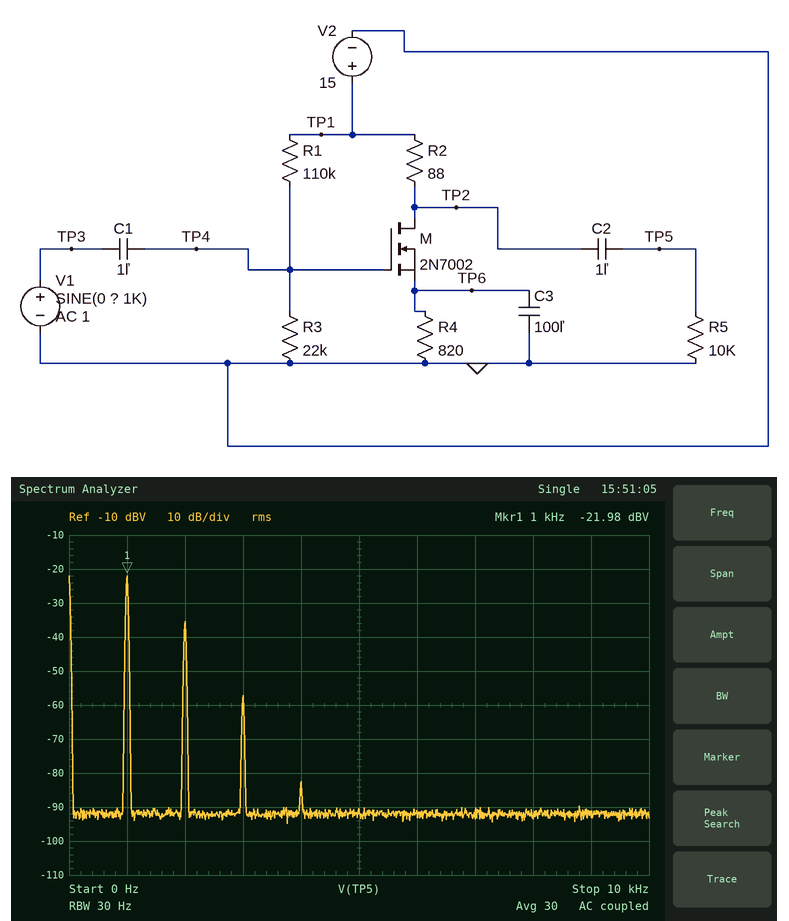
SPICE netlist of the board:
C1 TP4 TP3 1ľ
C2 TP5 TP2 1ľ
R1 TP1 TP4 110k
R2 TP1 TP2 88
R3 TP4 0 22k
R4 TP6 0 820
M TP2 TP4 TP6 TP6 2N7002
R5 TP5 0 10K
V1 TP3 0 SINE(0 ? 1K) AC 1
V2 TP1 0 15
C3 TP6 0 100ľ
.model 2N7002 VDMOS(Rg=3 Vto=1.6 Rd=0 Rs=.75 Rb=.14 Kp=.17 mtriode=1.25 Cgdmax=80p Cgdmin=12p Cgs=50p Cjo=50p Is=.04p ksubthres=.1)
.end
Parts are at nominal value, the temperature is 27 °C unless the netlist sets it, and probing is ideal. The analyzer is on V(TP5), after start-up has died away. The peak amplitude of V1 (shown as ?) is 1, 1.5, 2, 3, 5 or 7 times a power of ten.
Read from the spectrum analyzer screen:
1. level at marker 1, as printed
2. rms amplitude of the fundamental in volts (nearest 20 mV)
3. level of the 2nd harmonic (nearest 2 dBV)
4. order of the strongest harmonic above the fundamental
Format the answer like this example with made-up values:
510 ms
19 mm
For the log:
-21.98 dBV
80 mV
-36 dBV
2
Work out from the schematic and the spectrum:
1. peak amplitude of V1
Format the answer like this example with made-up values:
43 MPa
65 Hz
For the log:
100 mV
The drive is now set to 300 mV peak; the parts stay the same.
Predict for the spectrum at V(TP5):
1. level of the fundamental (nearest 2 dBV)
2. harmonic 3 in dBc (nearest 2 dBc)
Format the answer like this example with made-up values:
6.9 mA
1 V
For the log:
-10 dBV
-22 dBc
